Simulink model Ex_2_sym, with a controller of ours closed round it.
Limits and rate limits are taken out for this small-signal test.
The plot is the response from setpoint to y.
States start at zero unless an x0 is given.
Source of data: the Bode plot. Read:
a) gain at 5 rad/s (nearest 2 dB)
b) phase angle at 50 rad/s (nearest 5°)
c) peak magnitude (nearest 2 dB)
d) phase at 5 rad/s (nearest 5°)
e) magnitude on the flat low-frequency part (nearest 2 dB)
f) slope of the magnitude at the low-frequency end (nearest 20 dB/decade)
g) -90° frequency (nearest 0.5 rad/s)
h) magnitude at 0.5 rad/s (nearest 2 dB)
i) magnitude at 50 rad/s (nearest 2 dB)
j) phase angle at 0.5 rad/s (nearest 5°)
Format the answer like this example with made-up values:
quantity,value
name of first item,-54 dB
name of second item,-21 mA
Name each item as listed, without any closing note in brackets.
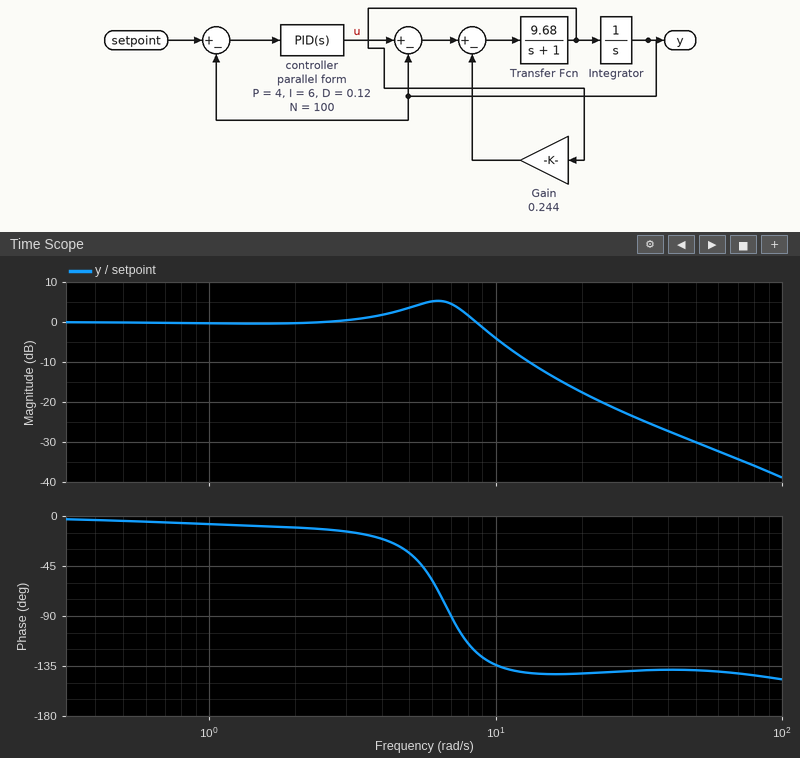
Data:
quantity,value
gain at 5 rad/s,4 dB
phase angle at 50 rad/s,-140°
peak magnitude,6 dB
phase at 5 rad/s,-35°
magnitude on the flat low-frequency part,0 dB
slope of the magnitude at the low-frequency end,0 dB/decade
-90° frequency,7.0 rad/s
magnitude at 0.5 rad/s,0 dB
magnitude at 50 rad/s,-30 dB
phase angle at 0.5 rad/s,-5°
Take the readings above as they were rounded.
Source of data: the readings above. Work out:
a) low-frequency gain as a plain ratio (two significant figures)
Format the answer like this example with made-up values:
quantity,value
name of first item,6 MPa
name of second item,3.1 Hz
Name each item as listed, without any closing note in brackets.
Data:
quantity,value
low-frequency gain as a plain ratio,1.0
